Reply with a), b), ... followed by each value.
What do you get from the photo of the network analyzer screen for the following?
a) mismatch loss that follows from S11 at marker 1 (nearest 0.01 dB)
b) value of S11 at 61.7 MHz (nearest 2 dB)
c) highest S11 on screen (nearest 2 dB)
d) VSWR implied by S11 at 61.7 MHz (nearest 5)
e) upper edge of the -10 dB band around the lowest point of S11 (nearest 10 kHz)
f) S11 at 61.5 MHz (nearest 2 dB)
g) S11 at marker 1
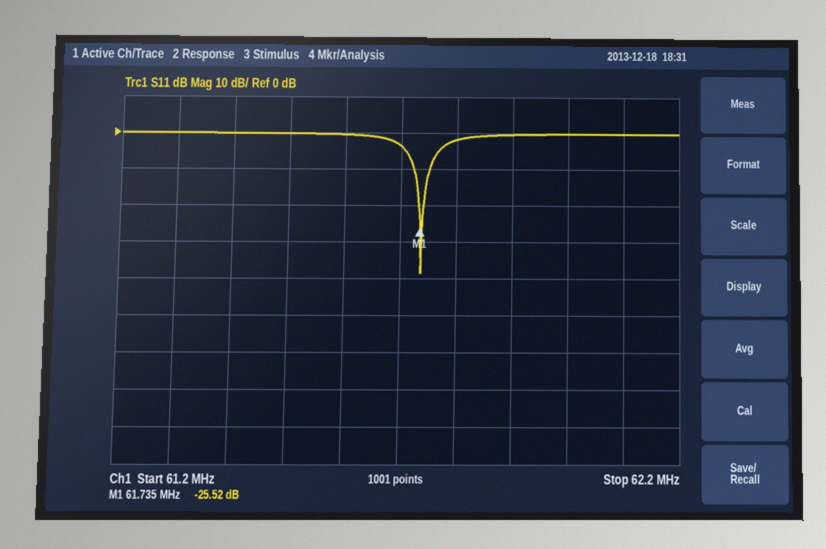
a) 0.01 dB
b) -4 dB
c) 0 dB
d) 5
e) 61.75 MHz
f) 0 dB
g) -25.52 dB
